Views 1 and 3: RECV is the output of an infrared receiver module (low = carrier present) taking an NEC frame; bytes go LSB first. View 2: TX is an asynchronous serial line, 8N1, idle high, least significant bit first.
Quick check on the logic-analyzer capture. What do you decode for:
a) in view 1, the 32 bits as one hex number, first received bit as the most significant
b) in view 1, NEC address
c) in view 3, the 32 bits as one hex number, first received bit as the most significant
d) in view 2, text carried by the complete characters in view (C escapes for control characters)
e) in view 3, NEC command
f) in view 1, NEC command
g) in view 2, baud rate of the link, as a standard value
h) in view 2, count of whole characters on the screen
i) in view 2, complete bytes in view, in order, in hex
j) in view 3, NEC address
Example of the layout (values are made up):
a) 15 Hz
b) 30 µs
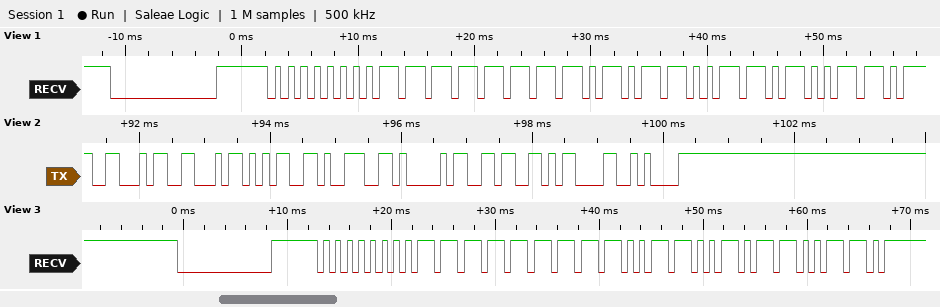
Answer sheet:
a) 0x00FF59A6
b) 0x00
c) 0x00FF9966
d) "FF59A6\r\n"
e) 0x99
f) 0x9A
g) 9600 baud
h) 8
i) 46 46 35 39 41 36 0D 0A
j) 0x00
